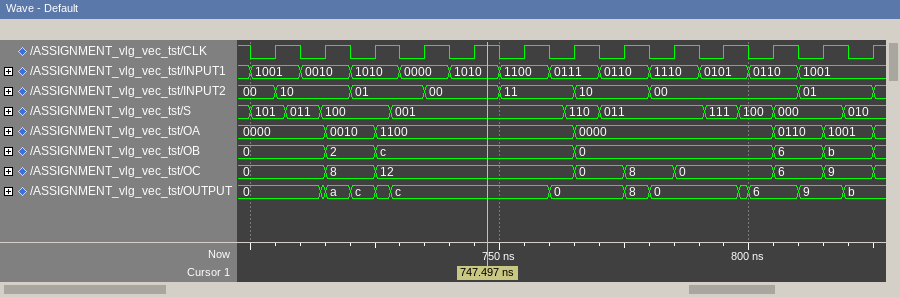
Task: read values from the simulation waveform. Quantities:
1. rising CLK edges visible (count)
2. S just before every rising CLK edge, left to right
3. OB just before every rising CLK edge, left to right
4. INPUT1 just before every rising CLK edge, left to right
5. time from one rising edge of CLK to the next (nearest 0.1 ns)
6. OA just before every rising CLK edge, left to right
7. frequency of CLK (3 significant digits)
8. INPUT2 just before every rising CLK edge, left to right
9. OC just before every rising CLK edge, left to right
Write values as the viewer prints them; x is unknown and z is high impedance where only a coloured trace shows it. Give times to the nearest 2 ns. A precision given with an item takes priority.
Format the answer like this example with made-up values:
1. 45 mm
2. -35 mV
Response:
1. 13
2. 101, 100, 100, 001, 001, 001, 110, 011, 011, 111, 100, 000, 010
3. 0, 0, 2, c, c, c, c, 0, 0, 0, 0, 6, b
4. 1001, 0010, 1010, 0000, 1010, 1100, 0111, 0110, 1110, 0101, 0110, 1001, 1001
5. 10 ns
6. 0000, 0000, 0010, 1100, 1100, 1100, 1100, 0000, 0000, 0000, 0000, 0110, 1001
7. 100 MHz
8. 00, 10, 01, 01, 00, 11, 11, 10, 00, 00, 00, 01, 01
9. 0, 0, 8, 12, 12, 12, 12, 0, 8, 0, 0, 6, 9
